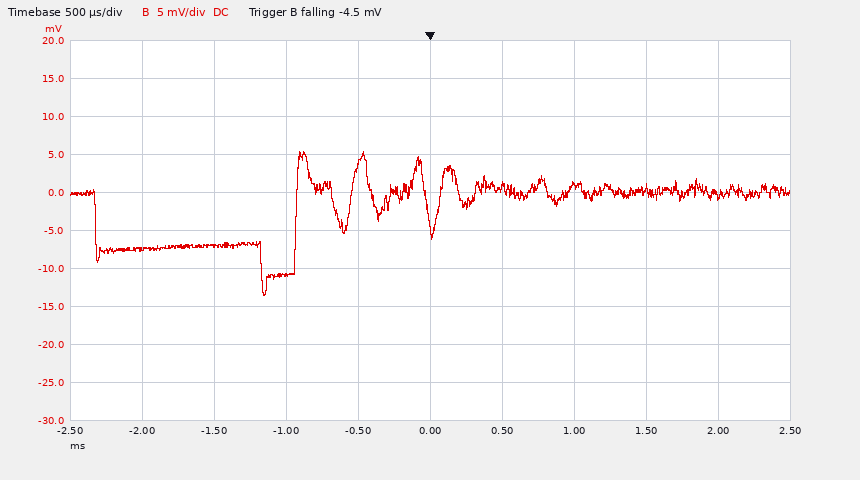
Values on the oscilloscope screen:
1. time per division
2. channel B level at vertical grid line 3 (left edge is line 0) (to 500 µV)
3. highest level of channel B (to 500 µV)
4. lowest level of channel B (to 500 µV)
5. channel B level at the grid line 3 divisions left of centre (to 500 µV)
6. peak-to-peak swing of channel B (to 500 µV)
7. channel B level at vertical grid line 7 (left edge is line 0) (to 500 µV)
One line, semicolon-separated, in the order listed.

500 µs; -11.0 mV; 5.5 mV; -13.5 mV; -7.0 mV; 19.0 mV; 1.0 mV
